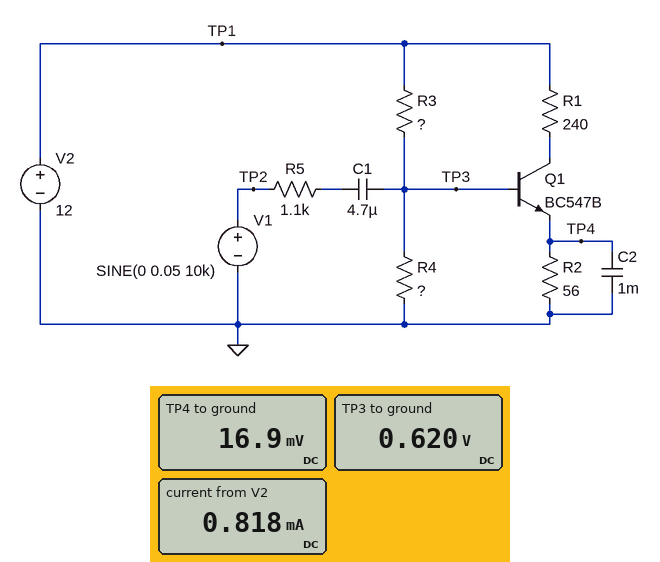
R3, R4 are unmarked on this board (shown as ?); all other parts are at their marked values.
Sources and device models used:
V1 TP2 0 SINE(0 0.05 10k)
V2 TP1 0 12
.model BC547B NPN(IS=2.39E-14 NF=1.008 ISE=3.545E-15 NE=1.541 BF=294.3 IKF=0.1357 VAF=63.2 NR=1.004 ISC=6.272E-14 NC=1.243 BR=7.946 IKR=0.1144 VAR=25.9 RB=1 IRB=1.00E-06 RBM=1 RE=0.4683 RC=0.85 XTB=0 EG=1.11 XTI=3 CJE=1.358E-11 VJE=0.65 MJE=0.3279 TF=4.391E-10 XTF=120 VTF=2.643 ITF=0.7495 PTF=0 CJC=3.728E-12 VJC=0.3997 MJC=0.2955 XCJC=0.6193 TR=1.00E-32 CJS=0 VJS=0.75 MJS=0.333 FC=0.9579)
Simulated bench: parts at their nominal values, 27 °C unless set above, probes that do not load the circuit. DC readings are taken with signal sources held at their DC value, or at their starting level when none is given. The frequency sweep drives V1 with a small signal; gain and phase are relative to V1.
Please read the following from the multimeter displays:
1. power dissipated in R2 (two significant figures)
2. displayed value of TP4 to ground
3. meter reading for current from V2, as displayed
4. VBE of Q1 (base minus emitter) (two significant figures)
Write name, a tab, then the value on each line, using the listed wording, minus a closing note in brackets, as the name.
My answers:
power dissipated in R2	5.1 µW
displayed value of TP4 to ground	16.9 mV
meter reading for current from V2, as displayed	0.818 mA
VBE of Q1 (base minus emitter)	600 mV
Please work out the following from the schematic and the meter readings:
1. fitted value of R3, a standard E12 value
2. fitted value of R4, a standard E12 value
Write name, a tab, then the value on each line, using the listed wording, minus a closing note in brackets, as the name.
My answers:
fitted value of R3, a standard E12 value	22 kΩ
fitted value of R4, a standard E12 value	1.2 kΩ
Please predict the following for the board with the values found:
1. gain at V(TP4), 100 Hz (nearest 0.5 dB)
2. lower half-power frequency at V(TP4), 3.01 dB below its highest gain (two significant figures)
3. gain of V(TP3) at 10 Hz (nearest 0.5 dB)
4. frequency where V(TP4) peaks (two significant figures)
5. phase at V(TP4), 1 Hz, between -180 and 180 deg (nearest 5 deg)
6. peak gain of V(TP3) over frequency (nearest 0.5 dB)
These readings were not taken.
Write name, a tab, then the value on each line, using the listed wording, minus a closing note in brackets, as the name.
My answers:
gain at V(TP4), 100 Hz	-41.0 dB
lower half-power frequency at V(TP4), 3.01 dB below its highest gain	3.1 Hz
gain of V(TP3) at 10 Hz	-11.5 dB
frequency where V(TP4) peaks	8.4 Hz
phase at V(TP4), 1 Hz, between -180 and 180 deg	75 deg
peak gain of V(TP3) over frequency	-6.0 dB
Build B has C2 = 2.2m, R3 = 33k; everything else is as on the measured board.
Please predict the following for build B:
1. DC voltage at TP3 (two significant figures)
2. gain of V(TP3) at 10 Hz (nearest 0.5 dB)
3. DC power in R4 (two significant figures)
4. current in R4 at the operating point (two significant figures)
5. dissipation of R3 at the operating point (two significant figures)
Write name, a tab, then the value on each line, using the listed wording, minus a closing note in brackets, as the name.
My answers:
DC voltage at TP3	420 mV
gain of V(TP3) at 10 Hz	-11.0 dB
DC power in R4	150 µW
current in R4 at the operating point	350 µA
dissipation of R3 at the operating point	4.1 mW
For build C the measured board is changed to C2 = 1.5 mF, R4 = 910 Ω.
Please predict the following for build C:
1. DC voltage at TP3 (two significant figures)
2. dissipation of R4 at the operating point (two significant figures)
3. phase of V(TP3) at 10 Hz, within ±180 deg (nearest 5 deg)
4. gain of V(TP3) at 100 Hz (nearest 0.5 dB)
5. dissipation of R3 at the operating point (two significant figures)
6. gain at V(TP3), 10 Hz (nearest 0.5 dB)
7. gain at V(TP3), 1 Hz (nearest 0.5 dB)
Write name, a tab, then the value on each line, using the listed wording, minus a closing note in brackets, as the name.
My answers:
DC voltage at TP3	480 mV
dissipation of R4 at the operating point	250 µW
phase of V(TP3) at 10 Hz, within ±180 deg	60 deg
gain of V(TP3) at 100 Hz	-7.0 dB
dissipation of R3 at the operating point	6.0 mW
gain at V(TP3), 10 Hz	-13.0 dB
gain at V(TP3), 1 Hz	-32.0 dB
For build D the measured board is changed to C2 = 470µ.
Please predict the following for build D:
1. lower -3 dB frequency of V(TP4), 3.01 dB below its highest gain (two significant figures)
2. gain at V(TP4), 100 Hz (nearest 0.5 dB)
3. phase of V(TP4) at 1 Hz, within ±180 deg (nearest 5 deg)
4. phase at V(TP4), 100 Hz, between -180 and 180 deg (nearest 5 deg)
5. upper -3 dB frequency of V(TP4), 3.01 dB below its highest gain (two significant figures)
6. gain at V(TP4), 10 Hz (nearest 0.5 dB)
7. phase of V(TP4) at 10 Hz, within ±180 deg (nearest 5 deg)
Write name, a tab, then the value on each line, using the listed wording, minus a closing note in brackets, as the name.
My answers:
lower -3 dB frequency of V(TP4), 3.01 dB below its highest gain	5.0 Hz
gain at V(TP4), 100 Hz	-34.5 dB
phase of V(TP4) at 1 Hz, within ±180 deg	80 deg
phase at V(TP4), 100 Hz, between -180 and 180 deg	-75 deg
upper -3 dB frequency of V(TP4), 3.01 dB below its highest gain	30 Hz
gain at V(TP4), 10 Hz	-22.5 dB
phase of V(TP4) at 10 Hz, within ±180 deg	10 deg
